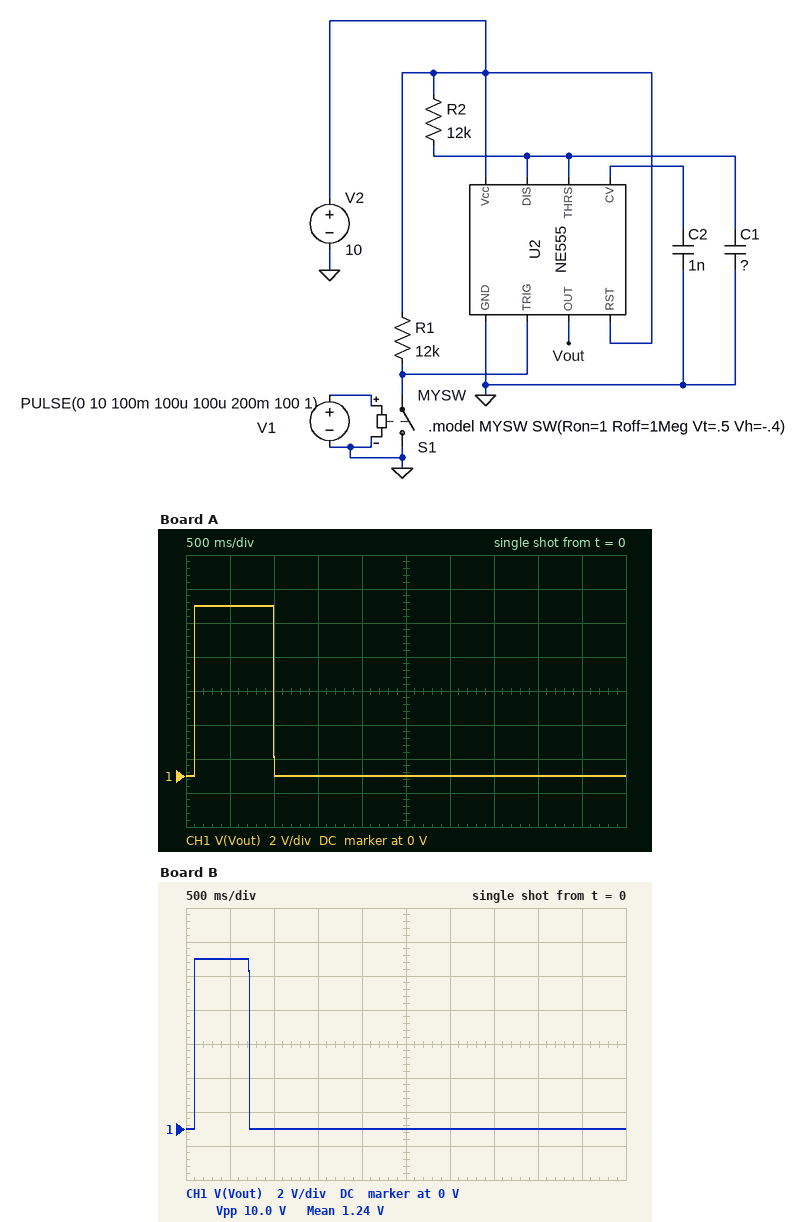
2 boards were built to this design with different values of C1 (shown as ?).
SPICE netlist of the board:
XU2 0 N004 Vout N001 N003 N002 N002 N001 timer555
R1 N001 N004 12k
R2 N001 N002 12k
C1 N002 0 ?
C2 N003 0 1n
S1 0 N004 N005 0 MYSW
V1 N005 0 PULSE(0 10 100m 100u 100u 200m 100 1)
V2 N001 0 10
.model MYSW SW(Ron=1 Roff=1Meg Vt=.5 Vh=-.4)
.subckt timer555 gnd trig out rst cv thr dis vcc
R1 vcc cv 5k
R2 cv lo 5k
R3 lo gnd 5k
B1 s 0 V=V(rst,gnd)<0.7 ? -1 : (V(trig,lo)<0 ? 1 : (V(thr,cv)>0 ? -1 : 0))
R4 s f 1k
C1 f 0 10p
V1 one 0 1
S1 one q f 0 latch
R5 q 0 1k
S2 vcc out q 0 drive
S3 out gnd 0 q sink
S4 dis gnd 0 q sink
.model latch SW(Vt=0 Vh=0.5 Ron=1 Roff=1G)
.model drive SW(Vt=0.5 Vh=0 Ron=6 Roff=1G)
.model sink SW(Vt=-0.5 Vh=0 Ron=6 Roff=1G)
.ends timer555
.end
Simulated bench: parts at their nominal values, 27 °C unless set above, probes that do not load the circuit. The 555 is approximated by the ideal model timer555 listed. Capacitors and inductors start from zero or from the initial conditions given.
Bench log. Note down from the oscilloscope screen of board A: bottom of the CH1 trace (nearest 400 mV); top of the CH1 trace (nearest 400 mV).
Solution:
0 V
10.0 V
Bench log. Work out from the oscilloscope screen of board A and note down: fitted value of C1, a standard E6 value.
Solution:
68 µF
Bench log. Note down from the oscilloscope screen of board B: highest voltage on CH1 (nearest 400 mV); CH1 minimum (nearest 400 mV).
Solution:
10.0 V
0 V
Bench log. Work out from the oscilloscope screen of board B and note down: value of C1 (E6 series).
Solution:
47 µF
